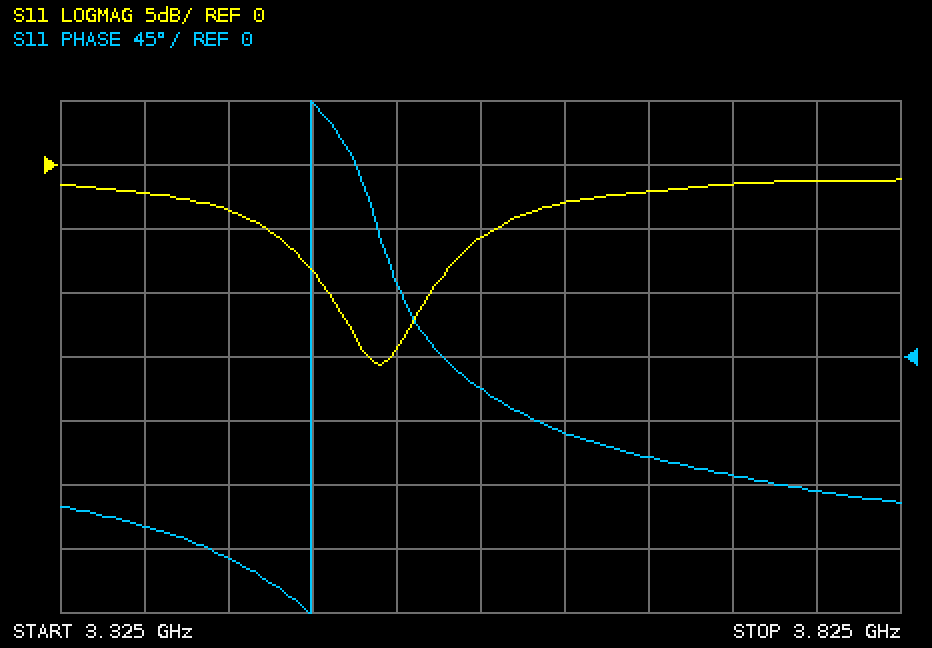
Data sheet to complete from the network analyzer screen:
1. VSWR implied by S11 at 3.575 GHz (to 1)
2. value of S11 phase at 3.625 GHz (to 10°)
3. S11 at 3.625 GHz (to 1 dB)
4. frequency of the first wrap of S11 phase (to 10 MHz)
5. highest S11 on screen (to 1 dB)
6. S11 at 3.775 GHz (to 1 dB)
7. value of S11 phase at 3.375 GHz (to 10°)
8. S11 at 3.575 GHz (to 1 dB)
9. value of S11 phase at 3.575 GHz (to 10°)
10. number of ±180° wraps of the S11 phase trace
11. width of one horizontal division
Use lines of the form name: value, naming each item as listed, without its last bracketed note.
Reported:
VSWR implied by S11 at 3.575 GHz: 3
value of S11 phase at 3.625 GHz: -50°
S11 at 3.625 GHz: -3 dB
frequency of the first wrap of S11 phase: 3.47 GHz
highest S11 on screen: -1 dB
S11 at 3.775 GHz: -1 dB
value of S11 phase at 3.375 GHz: -120°
S11 at 3.575 GHz: -6 dB
value of S11 phase at 3.575 GHz: -20°
number of ±180° wraps of the S11 phase trace: 1
width of one horizontal division: 50 MHz
